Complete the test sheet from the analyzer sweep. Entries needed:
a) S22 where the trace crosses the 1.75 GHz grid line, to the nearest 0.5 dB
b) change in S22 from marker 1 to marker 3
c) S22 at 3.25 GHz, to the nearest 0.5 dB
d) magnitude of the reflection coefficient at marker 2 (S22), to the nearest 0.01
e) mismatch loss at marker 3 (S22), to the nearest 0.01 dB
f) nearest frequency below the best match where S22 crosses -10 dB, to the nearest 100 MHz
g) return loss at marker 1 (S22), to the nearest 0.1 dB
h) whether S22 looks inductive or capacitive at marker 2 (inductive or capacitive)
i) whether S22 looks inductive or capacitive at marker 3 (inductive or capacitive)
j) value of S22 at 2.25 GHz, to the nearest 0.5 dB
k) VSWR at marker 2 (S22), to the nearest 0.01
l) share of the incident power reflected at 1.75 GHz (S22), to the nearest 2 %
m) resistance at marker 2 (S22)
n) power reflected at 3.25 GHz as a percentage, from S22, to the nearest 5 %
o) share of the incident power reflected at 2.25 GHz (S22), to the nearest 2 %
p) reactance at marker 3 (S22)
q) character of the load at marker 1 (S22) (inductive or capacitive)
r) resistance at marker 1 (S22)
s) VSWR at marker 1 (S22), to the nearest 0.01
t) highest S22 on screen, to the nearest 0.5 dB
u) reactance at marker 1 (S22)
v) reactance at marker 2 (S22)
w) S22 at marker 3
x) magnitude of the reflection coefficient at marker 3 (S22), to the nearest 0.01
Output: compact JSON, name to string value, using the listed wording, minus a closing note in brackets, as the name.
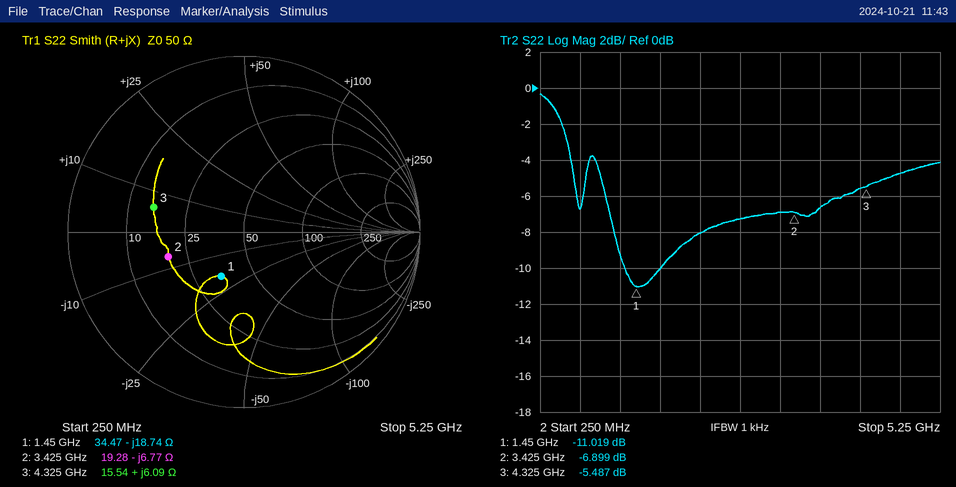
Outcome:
{"S22 where the trace crosses the 1.75 GHz grid line, to the nearest 0.5 dB": "-10.0 dB", "change in S22 from marker 1 to marker 3": "5.532 dB", "S22 at 3.25 GHz, to the nearest 0.5 dB": "-7.0 dB", "magnitude of the reflection coefficient at marker 2 (S22), to the nearest 0.01": "0.45", "mismatch loss at marker 3 (S22), to the nearest 0.01 dB": "1.44 dB", "nearest frequency below the best match where S22 crosses -10 dB, to the nearest 100 MHz": "1.3 GHz", "return loss at marker 1 (S22), to the nearest 0.1 dB": "11.0 dB", "whether S22 looks inductive or capacitive at marker 2": "capacitive", "whether S22 looks inductive or capacitive at marker 3": "inductive", "value of S22 at 2.25 GHz, to the nearest 0.5 dB": "-8.0 dB", "VSWR at marker 2 (S22), to the nearest 0.01": "2.65", "share of the incident power reflected at 1.75 GHz (S22), to the nearest 2 %": "10 %", "resistance at marker 2": "19.28 Ω", "power reflected at 3.25 GHz as a percentage, from S22, to the nearest 5 %": "20 %", "share of the incident power reflected at 2.25 GHz (S22), to the nearest 2 %": "16 %", "reactance at marker 3": "+6.09 Ω", "character of the load at marker 1 (S22)": "capacitive", "resistance at marker 1": "34.47 Ω", "VSWR at marker 1 (S22), to the nearest 0.01": "1.78", "highest S22 on screen, to the nearest 0.5 dB": "-0.5 dB", "reactance at marker 1": "-18.74 Ω", "reactance at marker 2": "-6.77 Ω", "S22 at marker 3": "-5.487 dB", "magnitude of the reflection coefficient at marker 3 (S22), to the nearest 0.01": "0.53"}
